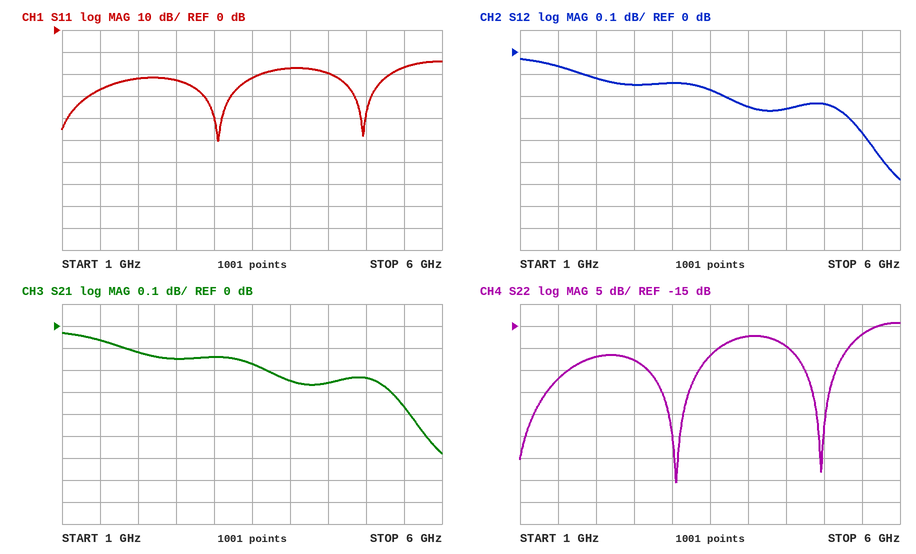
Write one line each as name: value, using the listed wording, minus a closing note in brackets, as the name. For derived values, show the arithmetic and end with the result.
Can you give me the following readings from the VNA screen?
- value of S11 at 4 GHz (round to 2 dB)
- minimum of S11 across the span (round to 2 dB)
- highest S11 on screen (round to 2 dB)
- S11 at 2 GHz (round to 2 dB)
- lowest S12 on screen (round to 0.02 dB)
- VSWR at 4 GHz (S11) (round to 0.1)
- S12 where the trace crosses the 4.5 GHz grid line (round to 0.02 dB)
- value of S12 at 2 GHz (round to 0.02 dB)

value of S11 at 4 GHz: -18 dB
minimum of S11 across the span: -50 dB
highest S11 on screen: -14 dB
S11 at 2 GHz: -22 dB
lowest S12 on screen: -0.58 dB
VSWR at 4 GHz (S11): |Γ| = 10^(-18/20) = 0.1259; VSWR = (1 + 0.1259)/(1 − 0.1259) ≈ 1.3
S12 where the trace crosses the 4.5 GHz grid line: -0.26 dB
value of S12 at 2 GHz: -0.12 dB
